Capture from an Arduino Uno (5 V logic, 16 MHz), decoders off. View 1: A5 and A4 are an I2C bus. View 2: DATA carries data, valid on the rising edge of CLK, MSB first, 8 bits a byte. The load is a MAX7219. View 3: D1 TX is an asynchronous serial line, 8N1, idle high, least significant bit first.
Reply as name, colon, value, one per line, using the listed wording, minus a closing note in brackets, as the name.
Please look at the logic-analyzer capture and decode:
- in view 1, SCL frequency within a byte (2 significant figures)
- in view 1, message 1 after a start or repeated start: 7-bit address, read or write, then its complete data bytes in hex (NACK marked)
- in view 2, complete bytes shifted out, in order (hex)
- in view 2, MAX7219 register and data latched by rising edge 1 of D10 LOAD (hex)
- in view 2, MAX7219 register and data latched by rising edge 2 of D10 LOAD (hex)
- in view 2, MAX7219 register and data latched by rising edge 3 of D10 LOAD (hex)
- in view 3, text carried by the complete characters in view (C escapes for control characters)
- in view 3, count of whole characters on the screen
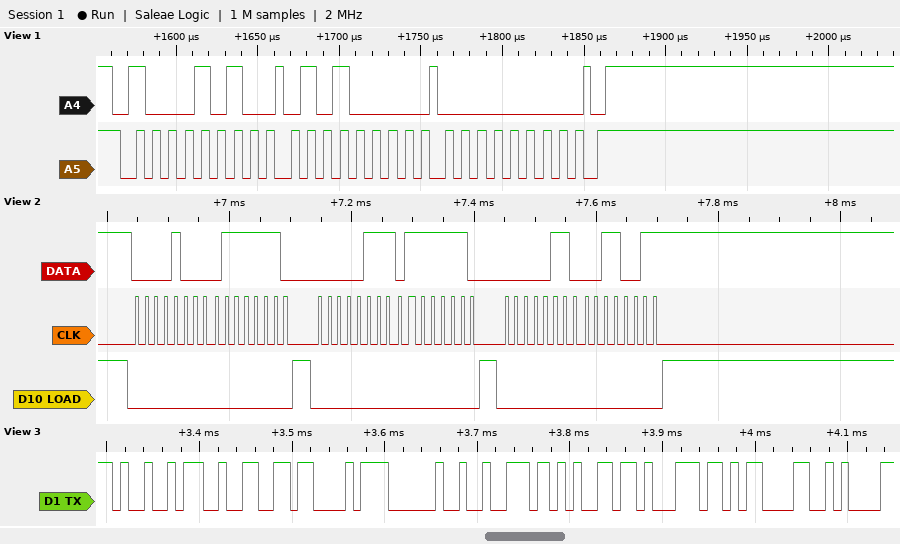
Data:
in view 1, SCL frequency within a byte: 100 kHz
in view 1, message 1 after a start or repeated start: 7-bit address, read or write, then its complete data bytes in hex: 0x45 write: 50 00
in view 2, complete bytes shifted out, in order: 08 7E 07 7E 06 33
in view 2, MAX7219 register and data latched by rising edge 1 of D10 LOAD: register 0x8, data 0x7E
in view 2, MAX7219 register and data latched by rising edge 2 of D10 LOAD: register 0x7, data 0x7E
in view 2, MAX7219 register and data latched by rising edge 3 of D10 LOAD: register 0x6, data 0x33
in view 3, text carried by the complete characters in view: "I2C req\r\n"
in view 3, count of whole characters on the screen: 9
